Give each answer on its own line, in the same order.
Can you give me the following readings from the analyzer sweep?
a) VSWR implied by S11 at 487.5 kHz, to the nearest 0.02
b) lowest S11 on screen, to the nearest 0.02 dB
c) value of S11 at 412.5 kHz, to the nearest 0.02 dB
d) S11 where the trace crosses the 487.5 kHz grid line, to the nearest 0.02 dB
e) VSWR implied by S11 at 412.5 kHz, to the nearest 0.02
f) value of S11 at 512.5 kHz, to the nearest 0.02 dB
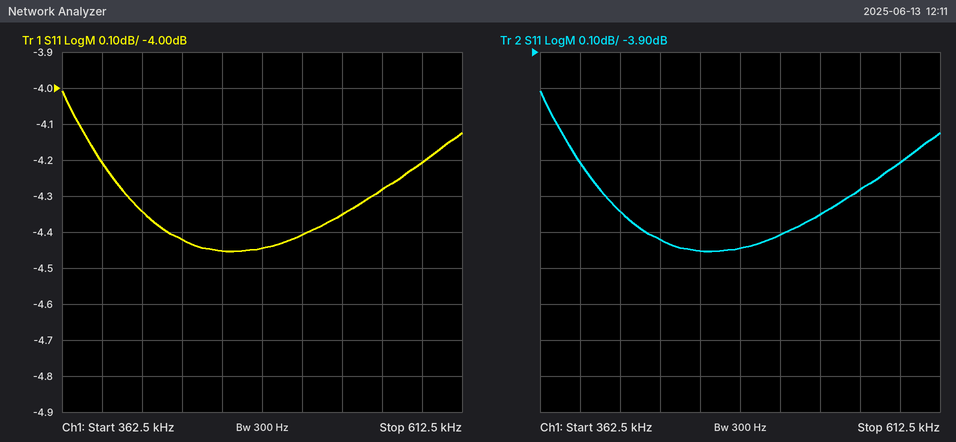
4.00
-4.46 dB
-4.34 dB
-4.44 dB
4.08
-4.40 dB
